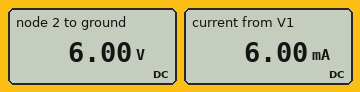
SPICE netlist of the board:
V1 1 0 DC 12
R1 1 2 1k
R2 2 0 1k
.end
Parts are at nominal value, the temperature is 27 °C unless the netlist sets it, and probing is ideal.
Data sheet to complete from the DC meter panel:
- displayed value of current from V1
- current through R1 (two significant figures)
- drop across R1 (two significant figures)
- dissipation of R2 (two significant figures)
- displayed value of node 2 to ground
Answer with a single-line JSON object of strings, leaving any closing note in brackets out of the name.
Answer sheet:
{"displayed value of current from V1": "6.00 mA", "current through R1": "6.0 mA", "drop across R1": "6.0 V", "dissipation of R2": "36 mW", "displayed value of node 2 to ground": "6.00 V"}
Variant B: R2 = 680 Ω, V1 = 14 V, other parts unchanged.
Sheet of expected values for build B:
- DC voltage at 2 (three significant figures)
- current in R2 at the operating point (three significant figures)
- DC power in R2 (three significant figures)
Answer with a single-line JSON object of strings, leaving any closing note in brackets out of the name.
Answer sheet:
{"DC voltage at 2": "5.67 V", "current in R2 at the operating point": "8.33 mA", "DC power in R2": "47.2 mW"}
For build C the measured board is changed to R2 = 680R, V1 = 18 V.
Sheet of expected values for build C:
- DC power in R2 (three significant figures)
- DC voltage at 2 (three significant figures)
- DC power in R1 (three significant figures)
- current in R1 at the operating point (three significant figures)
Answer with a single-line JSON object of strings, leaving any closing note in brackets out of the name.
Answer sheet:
{"DC power in R2": "78.1 mW", "DC voltage at 2": "7.29 V", "DC power in R1": "115 mW", "current in R1 at the operating point": "10.7 mA"}
